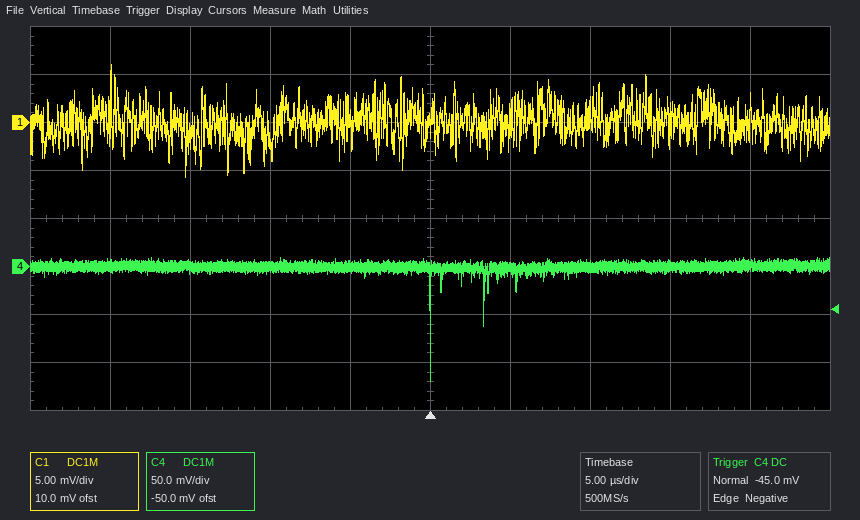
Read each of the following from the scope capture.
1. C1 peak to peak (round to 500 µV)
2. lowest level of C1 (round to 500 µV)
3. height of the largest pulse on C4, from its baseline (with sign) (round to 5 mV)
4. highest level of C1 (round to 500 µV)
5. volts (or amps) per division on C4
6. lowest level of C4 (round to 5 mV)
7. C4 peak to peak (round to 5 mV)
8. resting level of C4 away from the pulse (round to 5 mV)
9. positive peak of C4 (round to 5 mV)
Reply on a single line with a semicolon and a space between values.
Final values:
11.5 mV; -5.5 mV; -120 mV; 6.0 mV; 50 mV; -120 mV; 130 mV; 0 mV; 10 mV
